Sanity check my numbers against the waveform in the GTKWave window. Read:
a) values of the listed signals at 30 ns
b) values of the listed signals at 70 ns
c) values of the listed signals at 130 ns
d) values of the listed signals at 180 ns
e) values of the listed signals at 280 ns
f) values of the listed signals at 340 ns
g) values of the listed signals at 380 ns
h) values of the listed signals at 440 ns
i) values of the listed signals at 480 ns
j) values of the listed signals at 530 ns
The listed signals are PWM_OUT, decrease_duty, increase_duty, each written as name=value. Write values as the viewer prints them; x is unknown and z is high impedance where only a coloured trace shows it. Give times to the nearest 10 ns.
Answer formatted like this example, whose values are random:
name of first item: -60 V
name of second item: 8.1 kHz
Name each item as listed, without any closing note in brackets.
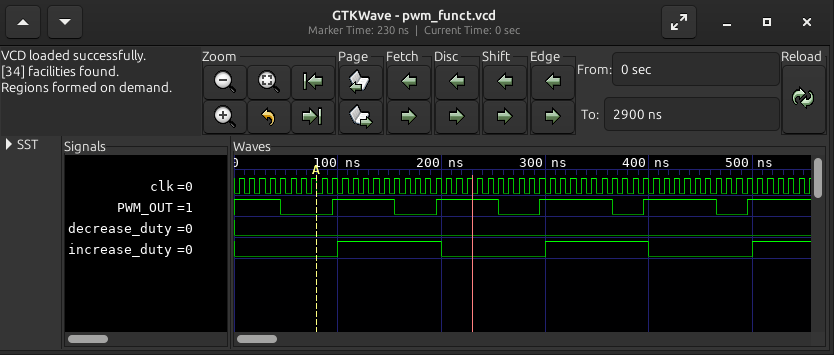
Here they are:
values of the listed signals at 30 ns: PWM_OUT=1, decrease_duty=0, increase_duty=0
values of the listed signals at 70 ns: PWM_OUT=0, decrease_duty=0, increase_duty=0
values of the listed signals at 130 ns: PWM_OUT=1, decrease_duty=0, increase_duty=1
values of the listed signals at 180 ns: PWM_OUT=0, decrease_duty=0, increase_duty=1
values of the listed signals at 280 ns: PWM_OUT=0, decrease_duty=0, increase_duty=0
values of the listed signals at 340 ns: PWM_OUT=1, decrease_duty=0, increase_duty=1
values of the listed signals at 380 ns: PWM_OUT=0, decrease_duty=0, increase_duty=1
values of the listed signals at 440 ns: PWM_OUT=1, decrease_duty=0, increase_duty=0
values of the listed signals at 480 ns: PWM_OUT=0, decrease_duty=0, increase_duty=0
values of the listed signals at 530 ns: PWM_OUT=1, decrease_duty=0, increase_duty=1
